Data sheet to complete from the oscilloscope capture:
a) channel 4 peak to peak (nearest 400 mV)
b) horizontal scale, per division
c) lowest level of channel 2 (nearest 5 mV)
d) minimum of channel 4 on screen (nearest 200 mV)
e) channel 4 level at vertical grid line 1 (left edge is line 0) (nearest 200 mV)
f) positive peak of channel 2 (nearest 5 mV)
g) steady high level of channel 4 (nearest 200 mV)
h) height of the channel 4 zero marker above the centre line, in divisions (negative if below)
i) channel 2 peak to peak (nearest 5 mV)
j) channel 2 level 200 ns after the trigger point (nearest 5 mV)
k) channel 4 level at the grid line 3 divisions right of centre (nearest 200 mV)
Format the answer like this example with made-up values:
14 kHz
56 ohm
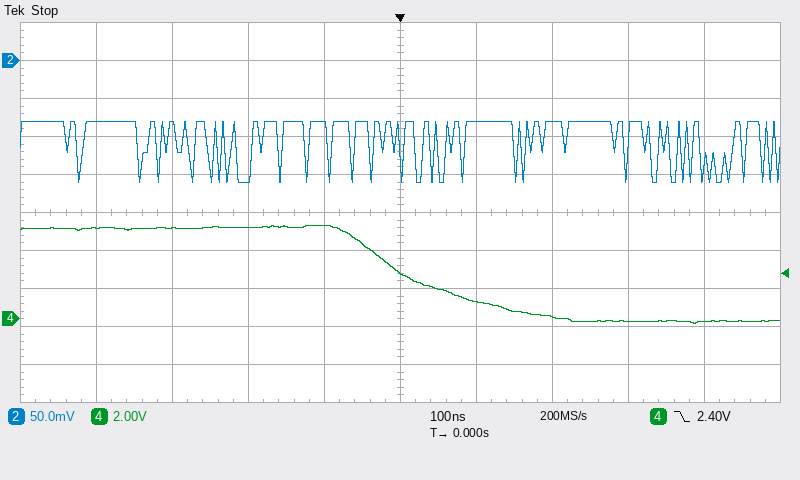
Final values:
5.2 V
100 ns
-160 mV
-200 mV
4.8 V
-80 mV
4.8 V
-2.8 div
80 mV
-80 mV
-200 mV
